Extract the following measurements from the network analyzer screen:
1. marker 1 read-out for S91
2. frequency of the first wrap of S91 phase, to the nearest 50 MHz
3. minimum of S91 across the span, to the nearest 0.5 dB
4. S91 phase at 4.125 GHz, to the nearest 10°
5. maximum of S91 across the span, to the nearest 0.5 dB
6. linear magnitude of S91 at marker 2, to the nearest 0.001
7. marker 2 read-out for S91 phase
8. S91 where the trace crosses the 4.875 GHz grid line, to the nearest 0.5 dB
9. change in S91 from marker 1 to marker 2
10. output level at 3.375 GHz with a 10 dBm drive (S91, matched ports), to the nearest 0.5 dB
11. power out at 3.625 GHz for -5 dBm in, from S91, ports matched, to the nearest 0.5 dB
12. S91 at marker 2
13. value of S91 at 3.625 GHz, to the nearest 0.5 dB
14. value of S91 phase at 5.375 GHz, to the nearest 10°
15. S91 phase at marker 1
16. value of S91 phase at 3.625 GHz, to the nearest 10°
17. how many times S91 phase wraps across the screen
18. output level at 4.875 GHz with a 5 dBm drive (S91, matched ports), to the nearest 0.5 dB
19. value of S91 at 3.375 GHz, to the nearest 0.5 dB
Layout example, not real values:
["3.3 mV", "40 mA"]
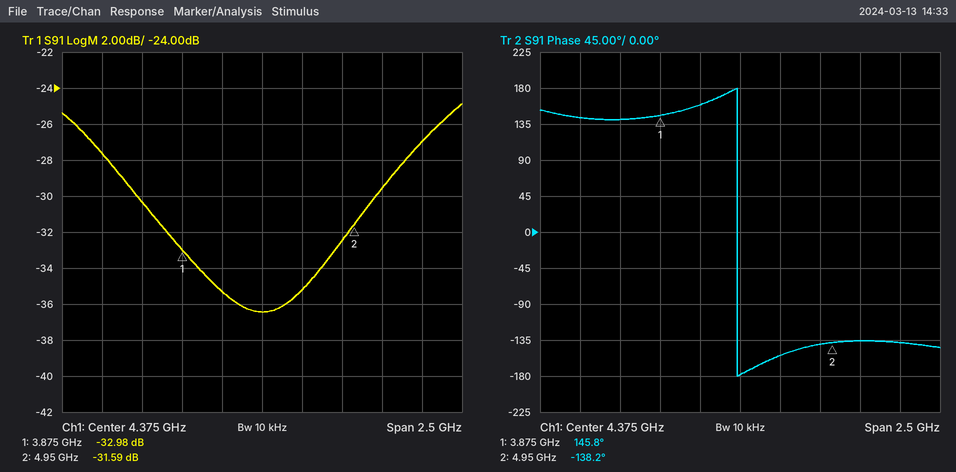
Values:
["-32.98 dB", "4.35 GHz", "-36.5 dB", "160°", "-25.0 dB", "0.026", "-138.2°", "-32.5 dB", "1.39 dB", "-17.5 dBm", "-35.5 dBm", "-31.59 dB", "-30.5 dB", "-140°", "145.8°", "140°", "1", "-27.5 dBm", "-27.5 dB"]
